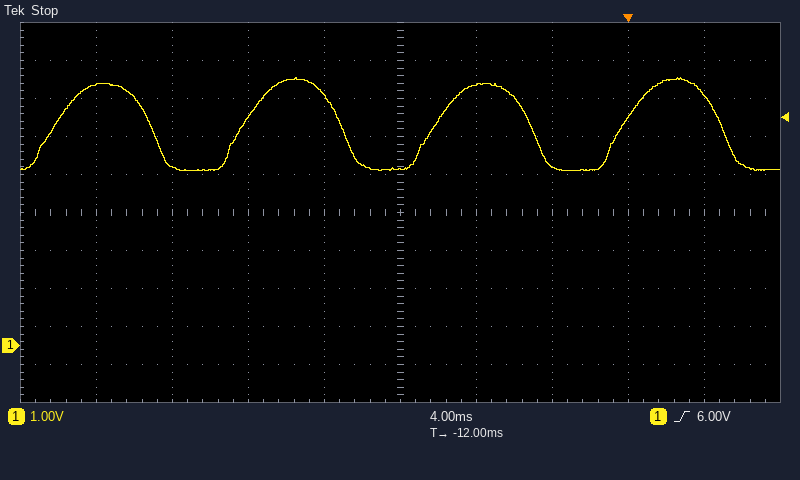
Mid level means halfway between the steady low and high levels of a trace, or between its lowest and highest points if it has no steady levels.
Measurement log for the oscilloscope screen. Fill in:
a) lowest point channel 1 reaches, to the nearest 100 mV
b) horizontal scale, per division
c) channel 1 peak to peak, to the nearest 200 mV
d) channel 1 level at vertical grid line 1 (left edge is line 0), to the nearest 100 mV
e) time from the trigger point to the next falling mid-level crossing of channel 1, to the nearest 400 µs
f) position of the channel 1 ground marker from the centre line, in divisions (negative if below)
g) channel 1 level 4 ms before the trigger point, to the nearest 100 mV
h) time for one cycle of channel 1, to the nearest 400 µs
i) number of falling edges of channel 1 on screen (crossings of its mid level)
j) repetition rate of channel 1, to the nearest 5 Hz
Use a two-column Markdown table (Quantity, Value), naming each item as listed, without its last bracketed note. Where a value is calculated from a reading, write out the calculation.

| Quantity | Value |
|---|---|
| lowest point channel 1 reaches, to the nearest 100 mV | 4.6 V |
| horizontal scale, per division | 4 ms |
| channel 1 peak to peak, to the nearest 200 mV | 2.4 V |
| channel 1 level at vertical grid line 1 (left edge is line 0), to the nearest 100 mV | 6.9 V |
| time from the trigger point to the next falling mid-level crossing of channel 1, to the nearest 400 µs | 4.8 ms |
| position of the channel 1 ground marker from the centre line, in divisions | -3.5 div |
| channel 1 level 4 ms before the trigger point, to the nearest 100 mV | 4.7 V |
| time for one cycle of channel 1, to the nearest 400 µs | 10.0 ms |
| number of falling edges of channel 1 on screen | 4 |
| repetition rate of channel 1, to the nearest 5 Hz | 1 / 10.0 ms ≈ 100 Hz |
